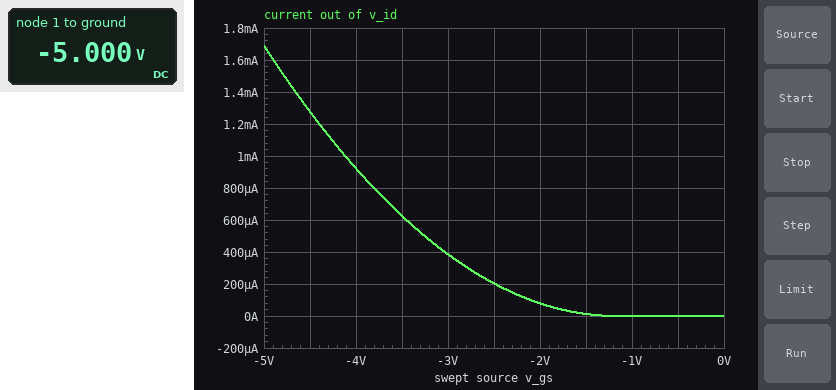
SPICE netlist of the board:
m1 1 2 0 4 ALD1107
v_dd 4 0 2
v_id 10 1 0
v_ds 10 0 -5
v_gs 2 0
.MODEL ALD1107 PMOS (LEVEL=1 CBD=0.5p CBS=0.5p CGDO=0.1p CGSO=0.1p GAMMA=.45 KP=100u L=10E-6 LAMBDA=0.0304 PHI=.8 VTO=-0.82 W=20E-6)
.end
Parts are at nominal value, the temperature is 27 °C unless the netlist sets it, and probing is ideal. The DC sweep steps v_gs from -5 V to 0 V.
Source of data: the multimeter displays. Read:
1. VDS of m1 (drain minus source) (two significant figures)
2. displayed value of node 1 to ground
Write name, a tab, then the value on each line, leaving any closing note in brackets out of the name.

VDS of m1 (drain minus source)	-5.0 V
displayed value of node 1 to ground	-5.000 V
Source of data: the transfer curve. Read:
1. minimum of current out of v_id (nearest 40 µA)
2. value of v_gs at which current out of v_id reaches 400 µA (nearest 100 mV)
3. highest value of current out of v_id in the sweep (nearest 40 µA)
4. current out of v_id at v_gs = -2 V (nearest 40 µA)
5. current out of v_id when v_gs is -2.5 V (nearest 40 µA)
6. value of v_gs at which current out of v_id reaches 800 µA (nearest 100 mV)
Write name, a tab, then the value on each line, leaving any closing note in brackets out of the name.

minimum of current out of v_id	0 A
value of v_gs at which current out of v_id reaches 400 µA	-3.0 V
highest value of current out of v_id in the sweep	1.68 mA
current out of v_id at v_gs = -2 V	80 µA
current out of v_id when v_gs is -2.5 V	200 µA
value of v_gs at which current out of v_id reaches 800 µA	-3.8 V
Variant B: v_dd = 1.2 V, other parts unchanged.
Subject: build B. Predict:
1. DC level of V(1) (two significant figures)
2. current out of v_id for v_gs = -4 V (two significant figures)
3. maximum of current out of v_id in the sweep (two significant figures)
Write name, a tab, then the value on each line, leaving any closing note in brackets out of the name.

DC level of V(1)	-5.0 V
current out of v_id for v_gs = -4 V	1.0 mA
maximum of current out of v_id in the sweep	1.8 mA
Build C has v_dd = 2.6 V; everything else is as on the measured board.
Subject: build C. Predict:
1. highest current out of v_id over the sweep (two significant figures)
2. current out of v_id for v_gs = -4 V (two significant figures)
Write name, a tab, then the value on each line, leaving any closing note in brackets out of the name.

highest current out of v_id over the sweep	1.6 mA
current out of v_id for v_gs = -4 V	870 µA
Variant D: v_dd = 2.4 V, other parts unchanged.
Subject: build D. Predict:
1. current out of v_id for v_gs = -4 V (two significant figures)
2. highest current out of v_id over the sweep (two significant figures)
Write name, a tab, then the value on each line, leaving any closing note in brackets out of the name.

current out of v_id for v_gs = -4 V	890 µA
highest current out of v_id over the sweep	1.6 mA
